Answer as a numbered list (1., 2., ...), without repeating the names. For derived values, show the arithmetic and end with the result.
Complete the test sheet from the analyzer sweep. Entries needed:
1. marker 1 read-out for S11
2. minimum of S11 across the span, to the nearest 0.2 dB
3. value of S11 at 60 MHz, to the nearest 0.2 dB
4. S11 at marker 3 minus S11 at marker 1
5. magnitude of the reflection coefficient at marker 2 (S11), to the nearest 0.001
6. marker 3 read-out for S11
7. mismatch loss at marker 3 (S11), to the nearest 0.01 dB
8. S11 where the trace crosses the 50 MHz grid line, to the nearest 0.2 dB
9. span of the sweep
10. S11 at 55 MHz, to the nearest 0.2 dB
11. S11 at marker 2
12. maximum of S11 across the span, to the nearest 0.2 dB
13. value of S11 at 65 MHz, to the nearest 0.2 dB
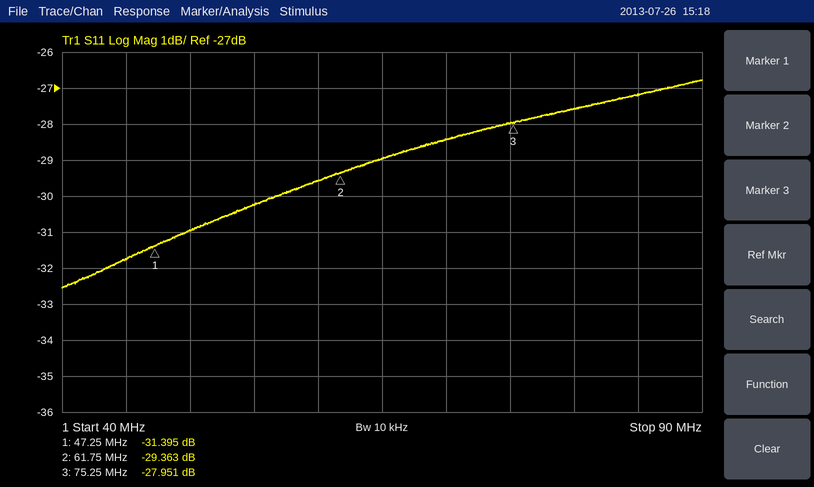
1. -31.395 dB
2. -32.6 dB
3. -29.6 dB
4. -27.951 − (-31.395) = 3.444 dB
5. 10^(-29.363/20) ≈ 0.034
6. -27.951 dB
7. −10 log10(1 − 10^(-27.951/10)) ≈ 0.01 dB
8. -31.0 dB
9. 50 MHz
10. -30.2 dB
11. -29.363 dB
12. -26.8 dB
13. -29.0 dB
